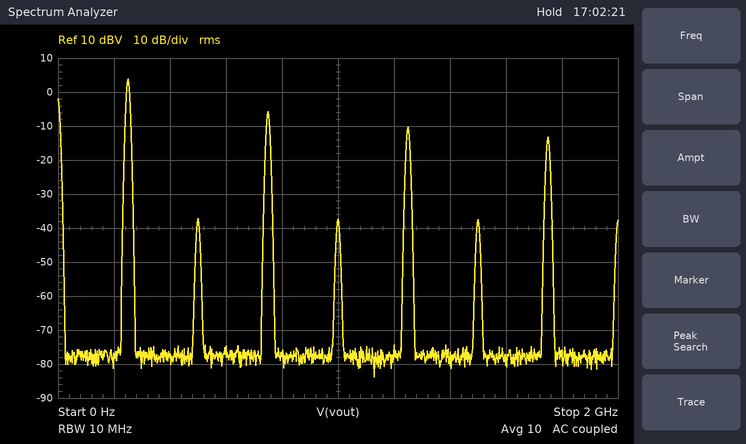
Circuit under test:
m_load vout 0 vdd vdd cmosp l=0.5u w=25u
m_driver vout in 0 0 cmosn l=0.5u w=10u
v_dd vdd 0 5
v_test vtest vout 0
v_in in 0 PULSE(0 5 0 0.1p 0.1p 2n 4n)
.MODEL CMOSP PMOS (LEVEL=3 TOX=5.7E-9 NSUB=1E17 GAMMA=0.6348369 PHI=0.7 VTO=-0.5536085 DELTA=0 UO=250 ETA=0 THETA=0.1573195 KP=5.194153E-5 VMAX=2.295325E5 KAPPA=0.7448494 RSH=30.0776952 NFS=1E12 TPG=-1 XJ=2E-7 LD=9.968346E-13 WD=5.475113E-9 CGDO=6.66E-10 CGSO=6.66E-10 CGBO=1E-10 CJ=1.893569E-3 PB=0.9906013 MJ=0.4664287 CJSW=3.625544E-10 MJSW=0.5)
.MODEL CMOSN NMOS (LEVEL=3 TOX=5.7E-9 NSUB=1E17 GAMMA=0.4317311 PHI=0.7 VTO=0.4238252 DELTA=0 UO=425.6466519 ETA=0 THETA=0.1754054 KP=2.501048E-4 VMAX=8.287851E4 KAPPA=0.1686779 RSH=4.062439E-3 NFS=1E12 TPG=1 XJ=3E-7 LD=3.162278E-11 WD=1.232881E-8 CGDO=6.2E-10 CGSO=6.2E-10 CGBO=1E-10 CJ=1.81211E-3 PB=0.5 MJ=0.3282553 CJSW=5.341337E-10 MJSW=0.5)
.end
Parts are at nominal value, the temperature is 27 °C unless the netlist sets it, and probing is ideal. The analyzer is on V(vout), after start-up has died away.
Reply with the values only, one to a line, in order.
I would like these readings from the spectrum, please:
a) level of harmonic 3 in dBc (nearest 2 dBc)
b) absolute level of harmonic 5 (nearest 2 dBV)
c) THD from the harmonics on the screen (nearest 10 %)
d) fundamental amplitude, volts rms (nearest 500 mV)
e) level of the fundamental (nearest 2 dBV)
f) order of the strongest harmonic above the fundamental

-10 dBc
-10 dBV
40 %
1.5 V
4 dBV
3
